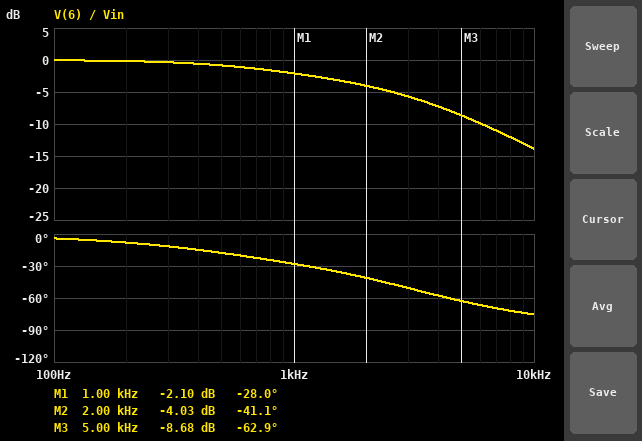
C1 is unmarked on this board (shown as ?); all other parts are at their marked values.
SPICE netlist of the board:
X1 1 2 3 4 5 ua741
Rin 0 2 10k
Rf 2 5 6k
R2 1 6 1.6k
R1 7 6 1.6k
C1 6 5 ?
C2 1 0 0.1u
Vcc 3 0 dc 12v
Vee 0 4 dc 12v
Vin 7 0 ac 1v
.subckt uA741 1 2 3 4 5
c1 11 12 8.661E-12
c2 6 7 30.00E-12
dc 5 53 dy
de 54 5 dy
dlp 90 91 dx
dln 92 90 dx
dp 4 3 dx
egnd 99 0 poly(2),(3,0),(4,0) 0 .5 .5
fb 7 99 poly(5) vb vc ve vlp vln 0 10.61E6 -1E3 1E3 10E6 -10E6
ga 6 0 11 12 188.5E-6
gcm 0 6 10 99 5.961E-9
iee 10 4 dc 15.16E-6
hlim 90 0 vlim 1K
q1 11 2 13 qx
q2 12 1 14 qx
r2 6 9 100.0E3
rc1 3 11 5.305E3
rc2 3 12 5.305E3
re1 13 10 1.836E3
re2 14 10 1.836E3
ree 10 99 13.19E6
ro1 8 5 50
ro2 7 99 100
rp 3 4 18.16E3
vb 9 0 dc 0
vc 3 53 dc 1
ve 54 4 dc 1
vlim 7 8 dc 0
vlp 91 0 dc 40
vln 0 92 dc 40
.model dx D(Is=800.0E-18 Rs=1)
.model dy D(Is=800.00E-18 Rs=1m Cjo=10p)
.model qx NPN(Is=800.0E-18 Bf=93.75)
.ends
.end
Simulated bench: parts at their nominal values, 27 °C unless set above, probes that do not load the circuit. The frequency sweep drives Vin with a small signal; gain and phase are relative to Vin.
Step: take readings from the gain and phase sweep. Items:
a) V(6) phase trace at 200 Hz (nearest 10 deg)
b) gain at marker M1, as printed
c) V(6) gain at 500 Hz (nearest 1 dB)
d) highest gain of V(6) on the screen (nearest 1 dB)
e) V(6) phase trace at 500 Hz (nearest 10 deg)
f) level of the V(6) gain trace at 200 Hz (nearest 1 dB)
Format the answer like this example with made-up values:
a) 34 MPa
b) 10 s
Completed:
a) -10 deg
b) -2.10 dB
c) -1 dB
d) 0 dB
e) -20 deg
f) 0 dB
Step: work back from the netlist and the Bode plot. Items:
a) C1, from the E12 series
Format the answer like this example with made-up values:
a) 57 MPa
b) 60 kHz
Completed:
a) 47 nF
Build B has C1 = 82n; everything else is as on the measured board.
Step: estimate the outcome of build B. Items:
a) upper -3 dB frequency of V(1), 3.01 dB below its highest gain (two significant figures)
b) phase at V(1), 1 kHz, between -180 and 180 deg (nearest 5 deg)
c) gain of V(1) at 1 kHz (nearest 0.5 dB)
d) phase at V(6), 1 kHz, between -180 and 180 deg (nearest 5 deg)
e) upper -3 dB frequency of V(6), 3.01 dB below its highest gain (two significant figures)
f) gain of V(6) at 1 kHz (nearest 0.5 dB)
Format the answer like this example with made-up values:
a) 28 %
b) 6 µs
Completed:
a) 910 Hz
b) -85 deg
c) -3.5 dB
d) -40 deg
e) 1.6 kHz
f) -0.5 dB
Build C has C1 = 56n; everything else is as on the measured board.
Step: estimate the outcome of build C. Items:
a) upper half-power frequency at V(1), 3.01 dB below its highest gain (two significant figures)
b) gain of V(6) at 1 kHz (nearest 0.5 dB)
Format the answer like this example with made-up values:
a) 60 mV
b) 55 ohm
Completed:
a) 740 Hz
b) -1.5 dB
